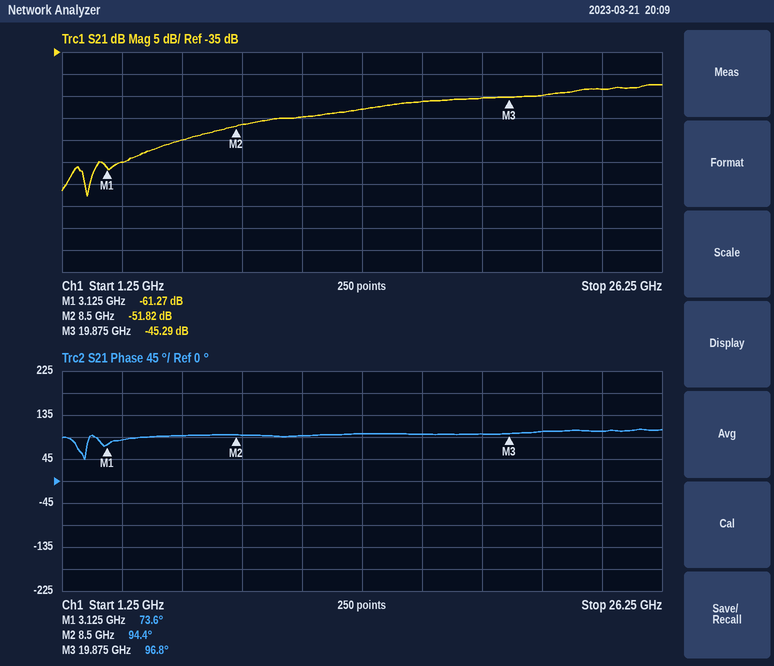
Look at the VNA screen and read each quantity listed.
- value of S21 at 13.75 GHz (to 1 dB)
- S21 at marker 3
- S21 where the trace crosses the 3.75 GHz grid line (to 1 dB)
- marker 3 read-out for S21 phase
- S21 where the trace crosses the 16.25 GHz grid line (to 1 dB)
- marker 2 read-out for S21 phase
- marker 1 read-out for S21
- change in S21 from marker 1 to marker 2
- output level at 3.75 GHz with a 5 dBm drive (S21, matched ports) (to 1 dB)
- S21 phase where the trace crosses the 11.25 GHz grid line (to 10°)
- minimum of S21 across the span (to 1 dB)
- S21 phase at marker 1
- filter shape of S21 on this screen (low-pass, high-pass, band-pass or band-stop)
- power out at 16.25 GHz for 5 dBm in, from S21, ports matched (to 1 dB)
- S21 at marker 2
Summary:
-48 dB
-45.29 dB
-60 dB
96.8°
-46 dB
94.4°
-61.27 dB
9.45 dB
-55 dBm
90°
-68 dB
73.6°
high-pass
-41 dBm
-51.82 dB
